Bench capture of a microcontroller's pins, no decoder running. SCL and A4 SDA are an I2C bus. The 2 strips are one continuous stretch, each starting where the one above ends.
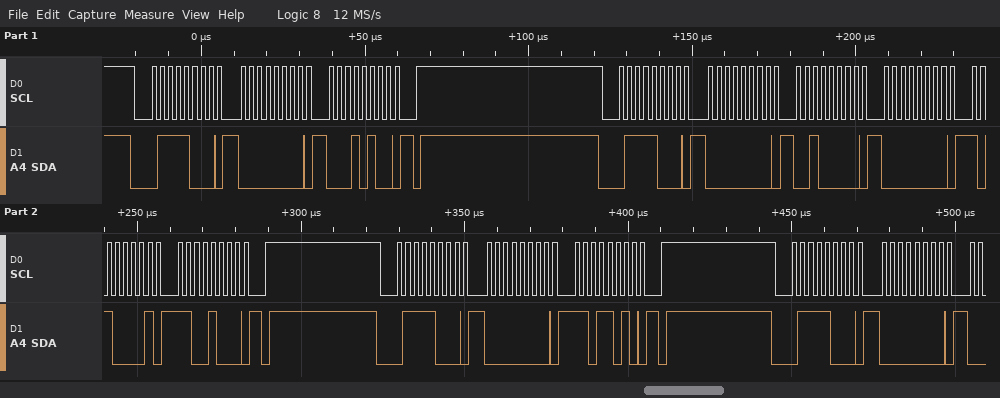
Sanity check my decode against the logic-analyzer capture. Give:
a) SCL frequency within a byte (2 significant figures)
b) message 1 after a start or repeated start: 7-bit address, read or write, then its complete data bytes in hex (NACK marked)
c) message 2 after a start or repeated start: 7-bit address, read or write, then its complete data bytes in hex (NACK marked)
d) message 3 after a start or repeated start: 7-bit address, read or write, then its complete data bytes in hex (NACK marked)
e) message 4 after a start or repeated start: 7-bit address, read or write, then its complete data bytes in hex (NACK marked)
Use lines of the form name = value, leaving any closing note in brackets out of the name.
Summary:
SCL frequency within a byte = 400 kHz
message 1 after a start or repeated start: 7-bit address, read or write, then its complete data bytes in hex = 0x3C write: 00 14
message 2 after a start or repeated start: 7-bit address, read or write, then its complete data bytes in hex = 0x3C write: 00 20 00 A1 C8
message 3 after a start or repeated start: 7-bit address, read or write, then its complete data bytes in hex = 0x3C write: 00 DA
message 4 after a start or repeated start: 7-bit address, read or write, then its complete data bytes in hex = 0x3C write: 00
